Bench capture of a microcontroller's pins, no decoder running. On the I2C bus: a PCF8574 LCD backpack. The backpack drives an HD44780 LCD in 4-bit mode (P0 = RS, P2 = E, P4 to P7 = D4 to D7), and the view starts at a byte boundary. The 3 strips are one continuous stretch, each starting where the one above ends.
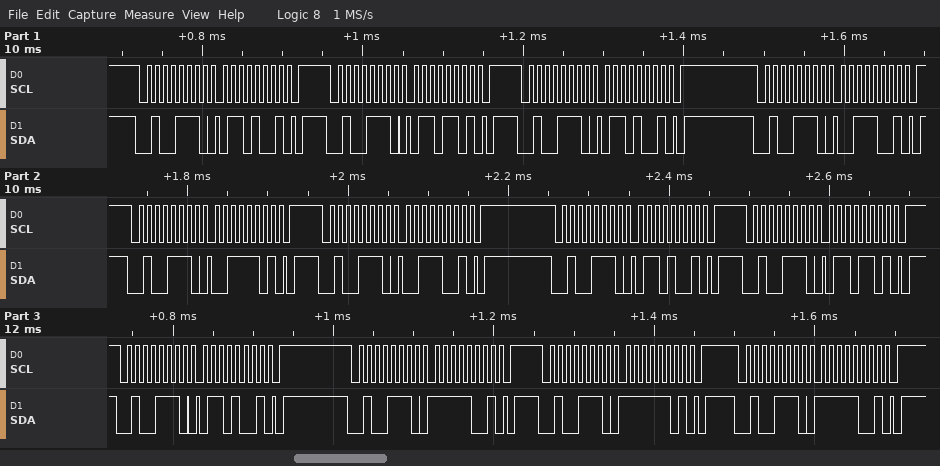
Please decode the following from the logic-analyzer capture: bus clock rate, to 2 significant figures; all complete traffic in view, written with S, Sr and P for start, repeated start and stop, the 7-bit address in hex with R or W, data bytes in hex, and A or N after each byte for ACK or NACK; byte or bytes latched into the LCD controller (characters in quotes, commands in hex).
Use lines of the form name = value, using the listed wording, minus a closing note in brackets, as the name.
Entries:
bus clock rate, to 2 significant figures = 100 kHz
all complete traffic in view, written with S, Sr and P for start, repeated start and stop, the 7-bit address in hex with R or W, data bytes in hex, and A or N after each byte for ACK or NACK = S 27W A 69 A P S 27W A 6D A P S 27W A 69 A P S 27W A 39 A P S 27W A 3D A P S 27W A 39 A P S 27W A 69 A P S 27W A 6D A P S 27W A 69 A P S 27W A F9 A P S 27W A FD A P S 27W A F9 A P
byte or bytes latched into the LCD controller = 'c' 'o'
